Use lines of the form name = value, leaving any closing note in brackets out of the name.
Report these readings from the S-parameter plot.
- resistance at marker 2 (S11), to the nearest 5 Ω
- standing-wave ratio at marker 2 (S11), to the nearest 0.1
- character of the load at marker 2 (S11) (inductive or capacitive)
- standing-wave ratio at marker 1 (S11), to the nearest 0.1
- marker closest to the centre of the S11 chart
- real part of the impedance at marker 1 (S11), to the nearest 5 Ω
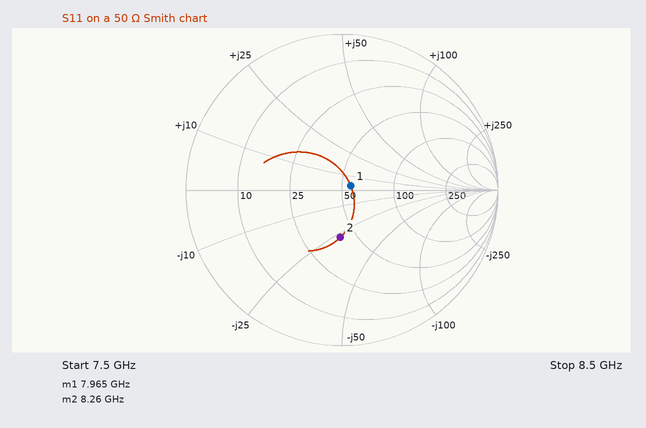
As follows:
resistance at marker 2 (S11), to the nearest 5 Ω = 40 Ω
standing-wave ratio at marker 2 (S11), to the nearest 0.1 = 1.9
character of the load at marker 2 (S11) = capacitive
standing-wave ratio at marker 1 (S11), to the nearest 0.1 = 1.1
marker closest to the centre of the S11 chart = marker 1
real part of the impedance at marker 1 (S11), to the nearest 5 Ω = 55 Ω
